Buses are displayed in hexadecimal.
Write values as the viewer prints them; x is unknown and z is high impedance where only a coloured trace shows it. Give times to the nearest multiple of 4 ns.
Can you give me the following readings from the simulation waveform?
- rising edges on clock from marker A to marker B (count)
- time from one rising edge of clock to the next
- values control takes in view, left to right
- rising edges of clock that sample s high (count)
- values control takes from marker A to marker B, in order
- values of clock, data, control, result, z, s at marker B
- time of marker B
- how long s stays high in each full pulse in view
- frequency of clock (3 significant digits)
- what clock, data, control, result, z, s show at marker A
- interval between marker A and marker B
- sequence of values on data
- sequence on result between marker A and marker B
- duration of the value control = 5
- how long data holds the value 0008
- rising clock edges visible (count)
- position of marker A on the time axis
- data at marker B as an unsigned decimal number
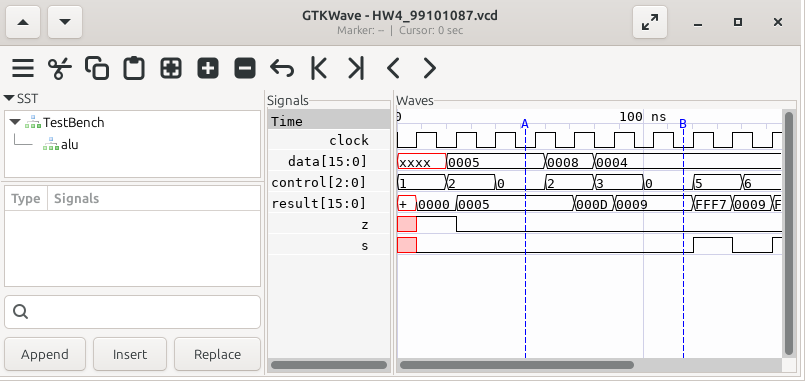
4
16 ns
1, 2, 0, 2, 3, 0, 5, 6
1
0, 2, 3, 0
clock=0, data=0004, control=0, result=0009, z=0, s=0
116 ns
16 ns
62.5 MHz
clock=0, data=0005, control=0, result=0005, z=0, s=0
64 ns
xxxx, 0005, 0008, 0004
0005, 000D, 0009
20 ns
20 ns
10
52 ns
4
